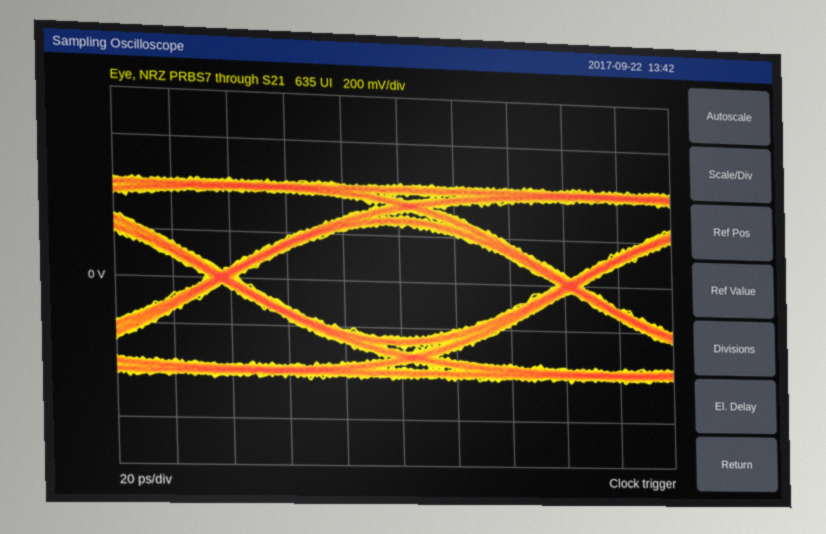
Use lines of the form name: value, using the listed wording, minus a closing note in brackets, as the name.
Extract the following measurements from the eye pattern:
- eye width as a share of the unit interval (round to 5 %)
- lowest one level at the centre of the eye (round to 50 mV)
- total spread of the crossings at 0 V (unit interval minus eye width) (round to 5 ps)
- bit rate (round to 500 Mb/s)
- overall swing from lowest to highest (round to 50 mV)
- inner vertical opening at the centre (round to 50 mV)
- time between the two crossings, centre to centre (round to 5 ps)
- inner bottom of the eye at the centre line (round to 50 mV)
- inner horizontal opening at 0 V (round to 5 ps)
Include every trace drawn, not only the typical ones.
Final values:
eye width as a share of the unit interval: 90 %
lowest one level at the centre of the eye: 250 mV
total spread of the crossings at 0 V (unit interval minus eye width): 10 ps
bit rate: 8.0 Gb/s
overall swing from lowest to highest: 850 mV
inner vertical opening at the centre: 500 mV
time between the two crossings, centre to centre: 125 ps
inner bottom of the eye at the centre line: -250 mV
inner horizontal opening at 0 V: 115 ps
